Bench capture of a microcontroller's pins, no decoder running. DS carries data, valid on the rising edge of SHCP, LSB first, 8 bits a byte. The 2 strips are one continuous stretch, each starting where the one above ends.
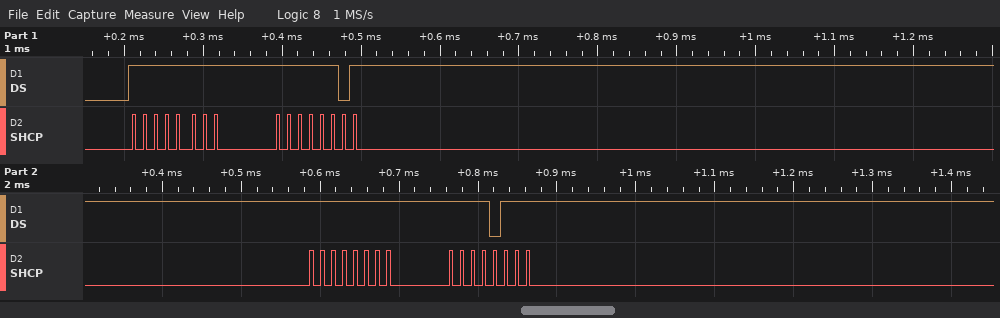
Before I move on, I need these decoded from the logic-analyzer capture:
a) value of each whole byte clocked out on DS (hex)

0xFF 0xBF 0xFF 0xEF
